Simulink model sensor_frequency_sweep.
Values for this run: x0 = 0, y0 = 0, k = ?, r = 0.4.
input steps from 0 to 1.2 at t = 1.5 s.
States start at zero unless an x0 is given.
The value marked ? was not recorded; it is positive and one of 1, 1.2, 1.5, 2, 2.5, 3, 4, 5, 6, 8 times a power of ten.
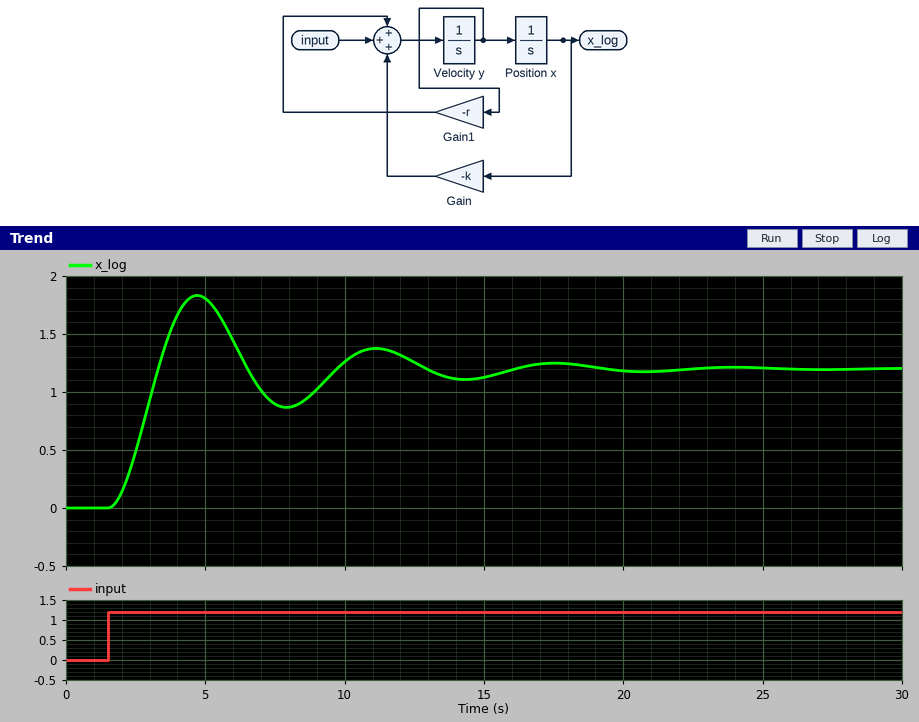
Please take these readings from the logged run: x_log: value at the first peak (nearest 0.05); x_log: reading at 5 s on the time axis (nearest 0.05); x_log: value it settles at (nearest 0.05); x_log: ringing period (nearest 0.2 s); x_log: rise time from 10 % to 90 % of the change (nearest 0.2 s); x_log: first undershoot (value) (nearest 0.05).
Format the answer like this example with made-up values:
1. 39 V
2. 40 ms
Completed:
1. 1.85
2. 1.80
3. 1.20
4. 6.4 s
5. 1.2 s
6. 0.85
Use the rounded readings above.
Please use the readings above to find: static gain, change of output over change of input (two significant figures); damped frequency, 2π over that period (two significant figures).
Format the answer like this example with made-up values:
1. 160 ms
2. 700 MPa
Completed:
1. 1.0
2. 0.98 rad/s
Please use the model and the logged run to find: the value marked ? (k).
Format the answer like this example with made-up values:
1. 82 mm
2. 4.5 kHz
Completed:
1. 1
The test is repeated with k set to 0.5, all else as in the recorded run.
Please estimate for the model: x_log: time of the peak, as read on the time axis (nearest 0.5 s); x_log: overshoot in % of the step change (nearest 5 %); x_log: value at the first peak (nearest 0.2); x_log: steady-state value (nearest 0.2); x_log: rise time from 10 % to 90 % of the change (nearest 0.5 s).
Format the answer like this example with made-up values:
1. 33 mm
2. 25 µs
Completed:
1. 6.0 s
2. 40 %
3. 3.4
4. 2.4
5. 2.0 s
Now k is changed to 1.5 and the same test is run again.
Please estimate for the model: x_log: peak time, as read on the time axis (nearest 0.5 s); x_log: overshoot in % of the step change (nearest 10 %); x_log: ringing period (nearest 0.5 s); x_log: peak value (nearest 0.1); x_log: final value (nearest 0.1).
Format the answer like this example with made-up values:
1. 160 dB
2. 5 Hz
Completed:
1. 4.0 s
2. 60 %
3. 5.0 s
4. 1.3
5. 0.8
